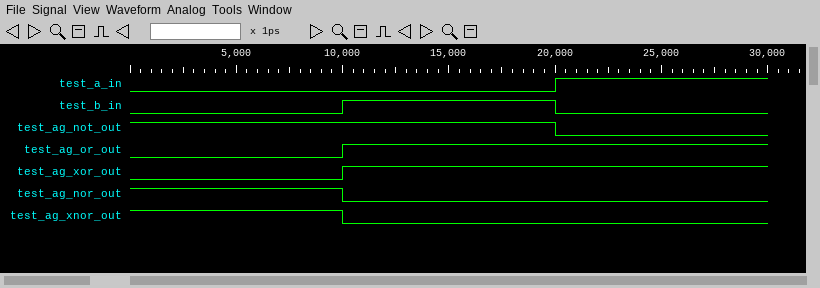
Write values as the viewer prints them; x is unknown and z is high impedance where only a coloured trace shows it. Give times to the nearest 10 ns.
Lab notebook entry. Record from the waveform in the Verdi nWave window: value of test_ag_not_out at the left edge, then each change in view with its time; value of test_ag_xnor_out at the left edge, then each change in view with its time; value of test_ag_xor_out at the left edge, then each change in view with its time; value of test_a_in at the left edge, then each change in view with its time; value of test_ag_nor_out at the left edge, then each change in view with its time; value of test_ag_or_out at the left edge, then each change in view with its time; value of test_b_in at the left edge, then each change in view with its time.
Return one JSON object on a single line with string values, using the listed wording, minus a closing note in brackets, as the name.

{"value of test_ag_not_out at the left edge, then each change in view with its time": "1, 0 at 20 ns", "value of test_ag_xnor_out at the left edge, then each change in view with its time": "1, 0 at 10 ns", "value of test_ag_xor_out at the left edge, then each change in view with its time": "0, 1 at 10 ns", "value of test_a_in at the left edge, then each change in view with its time": "0, 1 at 20 ns", "value of test_ag_nor_out at the left edge, then each change in view with its time": "1, 0 at 10 ns", "value of test_ag_or_out at the left edge, then each change in view with its time": "0, 1 at 10 ns", "value of test_b_in at the left edge, then each change in view with its time": "0, 1 at 10 ns, 0 at 20 ns"}
